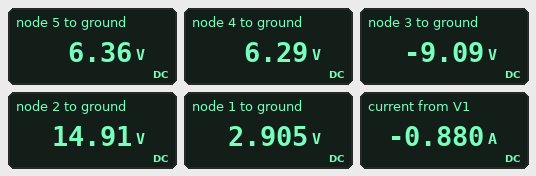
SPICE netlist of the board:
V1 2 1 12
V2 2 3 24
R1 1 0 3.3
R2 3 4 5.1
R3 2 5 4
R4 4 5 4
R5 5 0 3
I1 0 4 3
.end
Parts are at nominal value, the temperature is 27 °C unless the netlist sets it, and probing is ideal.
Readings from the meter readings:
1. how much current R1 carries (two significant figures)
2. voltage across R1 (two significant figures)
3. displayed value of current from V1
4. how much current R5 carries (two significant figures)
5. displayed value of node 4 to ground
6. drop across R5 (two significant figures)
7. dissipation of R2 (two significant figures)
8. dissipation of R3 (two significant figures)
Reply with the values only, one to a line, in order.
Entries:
880 mA
2.9 V
-0.880 A
2.1 A
6.29 V
6.4 V
46 W
18 W
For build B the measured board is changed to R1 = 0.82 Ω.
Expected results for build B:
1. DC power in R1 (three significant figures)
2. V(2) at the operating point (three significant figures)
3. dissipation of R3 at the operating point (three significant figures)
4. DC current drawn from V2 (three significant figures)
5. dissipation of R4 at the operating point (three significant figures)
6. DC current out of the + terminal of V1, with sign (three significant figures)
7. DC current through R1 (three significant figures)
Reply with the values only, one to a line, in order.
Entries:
1.20 W
13.0 V
14.5 W
3.12 A
55.6 mW
-1.21 A
1.21 A
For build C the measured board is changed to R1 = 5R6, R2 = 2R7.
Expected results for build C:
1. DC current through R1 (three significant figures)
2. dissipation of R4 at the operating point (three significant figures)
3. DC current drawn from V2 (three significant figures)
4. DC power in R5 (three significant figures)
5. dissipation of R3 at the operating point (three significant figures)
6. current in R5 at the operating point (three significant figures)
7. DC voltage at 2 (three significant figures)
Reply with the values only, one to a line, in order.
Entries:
942 mA
2.05 W
3.72 A
12.7 W
30.8 W
2.06 A
17.3 V
